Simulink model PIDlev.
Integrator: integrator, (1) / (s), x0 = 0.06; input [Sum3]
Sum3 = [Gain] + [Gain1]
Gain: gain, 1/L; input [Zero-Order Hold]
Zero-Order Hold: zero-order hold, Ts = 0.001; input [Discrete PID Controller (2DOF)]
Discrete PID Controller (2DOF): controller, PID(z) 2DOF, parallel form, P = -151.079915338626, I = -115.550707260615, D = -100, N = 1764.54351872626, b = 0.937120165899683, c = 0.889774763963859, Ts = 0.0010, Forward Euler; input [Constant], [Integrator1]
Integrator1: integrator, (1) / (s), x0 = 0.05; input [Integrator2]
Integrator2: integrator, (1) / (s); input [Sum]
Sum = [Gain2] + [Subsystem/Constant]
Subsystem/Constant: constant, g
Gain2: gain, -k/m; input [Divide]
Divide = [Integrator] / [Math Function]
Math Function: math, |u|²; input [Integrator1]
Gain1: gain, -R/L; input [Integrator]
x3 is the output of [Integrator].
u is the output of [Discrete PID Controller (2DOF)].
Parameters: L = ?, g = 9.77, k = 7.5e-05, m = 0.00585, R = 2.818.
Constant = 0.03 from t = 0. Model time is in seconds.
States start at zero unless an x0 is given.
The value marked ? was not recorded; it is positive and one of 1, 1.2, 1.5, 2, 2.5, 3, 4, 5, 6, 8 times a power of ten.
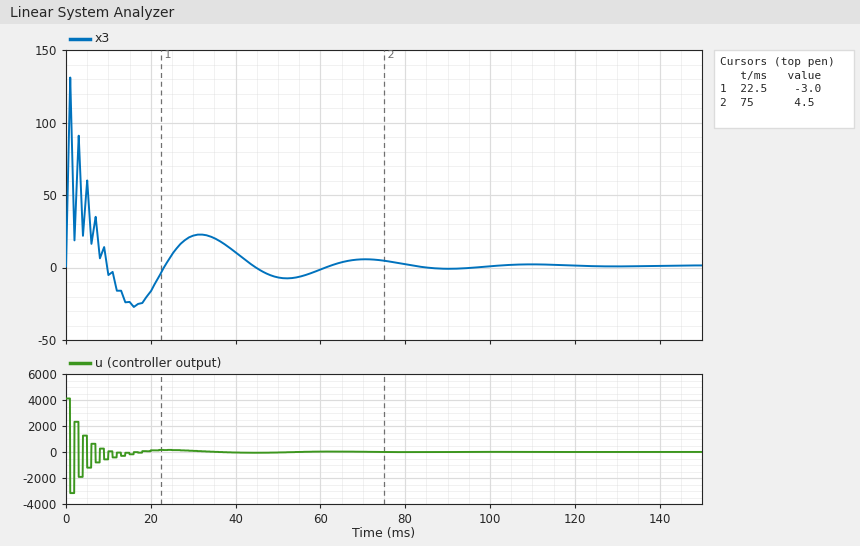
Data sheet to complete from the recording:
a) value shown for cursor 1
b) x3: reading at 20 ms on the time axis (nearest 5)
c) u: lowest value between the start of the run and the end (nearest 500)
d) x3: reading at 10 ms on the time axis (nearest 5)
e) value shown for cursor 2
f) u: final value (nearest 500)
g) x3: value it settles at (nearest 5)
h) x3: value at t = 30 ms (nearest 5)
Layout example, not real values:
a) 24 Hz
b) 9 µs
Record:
a) -3.0
b) -15
c) -3000
d) -5
e) 4.5
f) 0
g) 0
h) 20
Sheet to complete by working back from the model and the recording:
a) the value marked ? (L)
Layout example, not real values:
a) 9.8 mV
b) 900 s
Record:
a) 0.03
